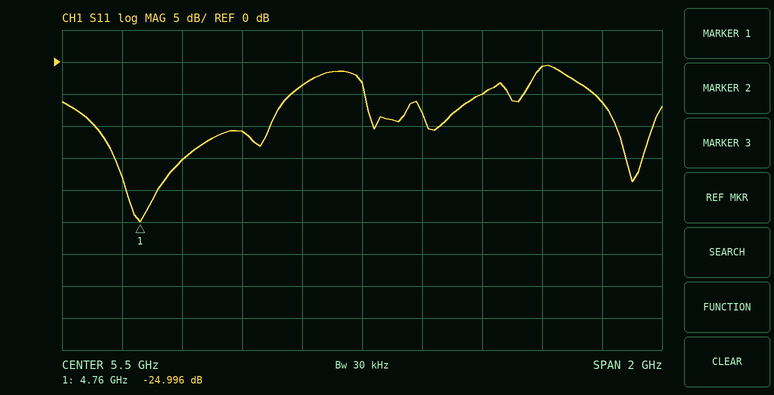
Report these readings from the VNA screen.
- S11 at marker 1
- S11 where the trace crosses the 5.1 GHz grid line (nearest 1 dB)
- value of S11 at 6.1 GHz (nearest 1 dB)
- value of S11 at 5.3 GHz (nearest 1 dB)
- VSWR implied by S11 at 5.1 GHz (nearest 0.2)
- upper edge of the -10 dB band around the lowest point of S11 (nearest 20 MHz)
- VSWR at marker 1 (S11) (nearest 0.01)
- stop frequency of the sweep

-24.996 dB
-11 dB
-1 dB
-4 dB
1.8
5.20 GHz
1.12
6.5 GHz
